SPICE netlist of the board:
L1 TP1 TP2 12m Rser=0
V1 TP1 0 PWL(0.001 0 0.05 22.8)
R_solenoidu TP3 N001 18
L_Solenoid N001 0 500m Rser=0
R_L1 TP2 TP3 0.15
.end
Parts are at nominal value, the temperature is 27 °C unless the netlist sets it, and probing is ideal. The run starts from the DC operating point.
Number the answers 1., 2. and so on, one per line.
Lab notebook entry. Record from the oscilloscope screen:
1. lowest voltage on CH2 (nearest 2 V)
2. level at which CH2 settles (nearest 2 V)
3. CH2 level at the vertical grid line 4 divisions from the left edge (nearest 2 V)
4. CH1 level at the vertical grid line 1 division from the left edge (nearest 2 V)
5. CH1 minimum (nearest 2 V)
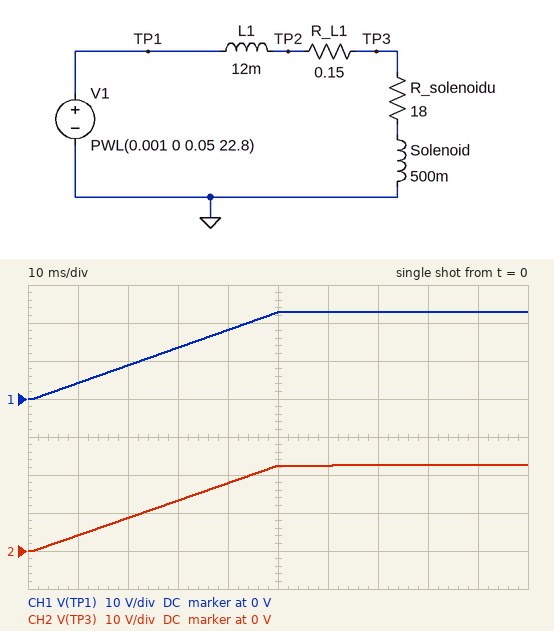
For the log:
1. 0 V
2. 22 V
3. 18 V
4. 4 V
5. 0 V
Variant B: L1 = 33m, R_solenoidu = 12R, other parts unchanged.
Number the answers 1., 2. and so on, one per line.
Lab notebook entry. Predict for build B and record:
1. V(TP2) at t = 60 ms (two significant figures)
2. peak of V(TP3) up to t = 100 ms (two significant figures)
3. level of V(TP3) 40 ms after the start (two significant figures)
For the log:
1. 22 V
2. 22 V
3. 17 V
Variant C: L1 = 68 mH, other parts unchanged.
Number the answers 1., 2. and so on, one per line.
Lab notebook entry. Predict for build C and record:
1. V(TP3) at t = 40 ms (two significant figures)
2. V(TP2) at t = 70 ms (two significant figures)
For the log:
1. 17 V
2. 22 V
